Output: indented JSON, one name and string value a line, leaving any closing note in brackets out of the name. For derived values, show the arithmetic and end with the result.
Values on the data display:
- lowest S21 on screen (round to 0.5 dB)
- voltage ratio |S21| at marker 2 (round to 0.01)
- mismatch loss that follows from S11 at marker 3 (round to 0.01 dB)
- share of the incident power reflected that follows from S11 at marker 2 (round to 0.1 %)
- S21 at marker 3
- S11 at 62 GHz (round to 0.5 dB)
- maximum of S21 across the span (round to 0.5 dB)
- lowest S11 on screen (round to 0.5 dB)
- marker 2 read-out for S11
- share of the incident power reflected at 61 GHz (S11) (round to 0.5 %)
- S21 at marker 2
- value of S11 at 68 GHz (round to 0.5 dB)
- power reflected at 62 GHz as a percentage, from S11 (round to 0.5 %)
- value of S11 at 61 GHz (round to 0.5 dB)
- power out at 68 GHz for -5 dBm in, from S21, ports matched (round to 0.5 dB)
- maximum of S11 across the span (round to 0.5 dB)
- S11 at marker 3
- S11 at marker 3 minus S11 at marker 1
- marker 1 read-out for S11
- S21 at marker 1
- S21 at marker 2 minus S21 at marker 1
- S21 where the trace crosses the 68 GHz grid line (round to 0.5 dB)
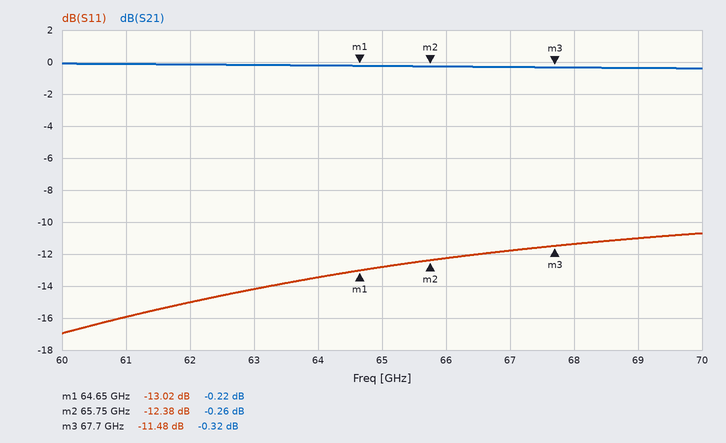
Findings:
{
  "lowest S21 on screen": "-0.5 dB",
  "voltage ratio |S21| at marker 2": "10^(-0.26/20) ≈ 0.97",
  "mismatch loss that follows from S11 at marker 3": "−10 log10(1 − 10^(-11.48/10)) ≈ 0.32 dB",
  "share of the incident power reflected that follows from S11 at marker 2": "10^(-12.38/10) ≈ 5.8 %",
  "S21 at marker 3": "-0.32 dB",
  "S11 at 62 GHz": "-15.0 dB",
  "maximum of S21 across the span": "0.0 dB",
  "lowest S11 on screen": "-17.0 dB",
  "marker 2 read-out for S11": "-12.38 dB",
  "share of the incident power reflected at 61 GHz (S11)": "10^(-16/10) ≈ 2.5 %",
  "S21 at marker 2": "-0.26 dB",
  "value of S11 at 68 GHz": "-11.5 dB",
  "power reflected at 62 GHz as a percentage, from S11": "10^(-15/10) ≈ 3.16 %, so 3.0 % to the nearest 0.5 %",
  "value of S11 at 61 GHz": "-16.0 dB",
  "power out at 68 GHz for -5 dBm in, from S21, ports matched": "-5 dBm + (-0.5 dB) = -5.5 dBm",
  "maximum of S11 across the span": "-10.5 dB",
  "S11 at marker 3": "-11.48 dB",
  "S11 at marker 3 minus S11 at marker 1": "-11.48 − (-13.02) = 1.54 dB",
  "marker 1 read-out for S11": "-13.02 dB",
  "S21 at marker 1": "-0.22 dB",
  "S21 at marker 2 minus S21 at marker 1": "-0.26 − (-0.22) = -0.04 dB",
  "S21 where the trace crosses the 68 GHz grid line": "-0.5 dB"
}
